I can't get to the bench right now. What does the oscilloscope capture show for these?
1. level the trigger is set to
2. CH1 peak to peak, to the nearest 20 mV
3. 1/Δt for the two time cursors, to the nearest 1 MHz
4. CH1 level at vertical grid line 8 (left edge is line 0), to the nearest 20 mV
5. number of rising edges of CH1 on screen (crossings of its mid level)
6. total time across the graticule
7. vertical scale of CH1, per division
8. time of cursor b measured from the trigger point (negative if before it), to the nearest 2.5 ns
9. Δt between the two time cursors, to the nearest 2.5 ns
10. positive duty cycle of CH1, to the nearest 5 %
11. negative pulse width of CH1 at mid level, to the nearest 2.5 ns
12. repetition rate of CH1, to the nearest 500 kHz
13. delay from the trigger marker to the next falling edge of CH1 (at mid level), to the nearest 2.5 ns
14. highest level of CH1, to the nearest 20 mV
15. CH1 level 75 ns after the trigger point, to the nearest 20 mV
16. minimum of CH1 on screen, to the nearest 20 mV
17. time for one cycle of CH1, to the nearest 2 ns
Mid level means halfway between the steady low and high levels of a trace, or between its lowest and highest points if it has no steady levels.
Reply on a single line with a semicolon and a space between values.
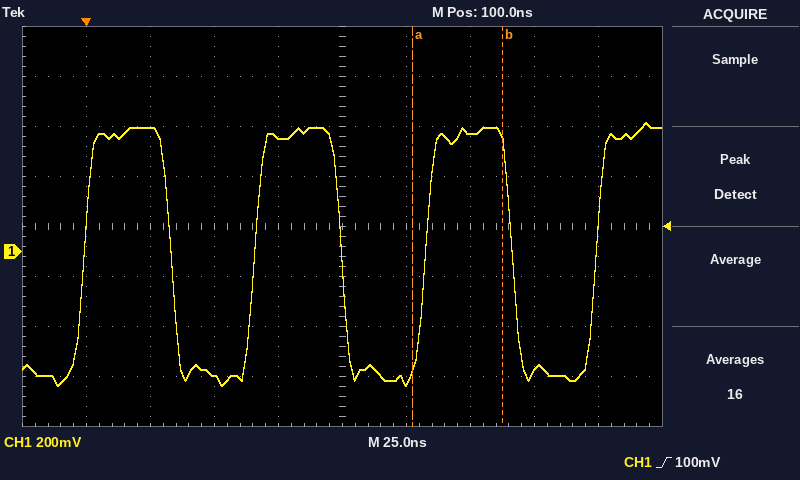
100 mV; 1.06 V; 29 MHz; -480 mV; 4; 250 ns; 200 mV; +162.5 ns; 35.0 ns; 50 %; 32.5 ns; 15.0 MHz; 32.5 ns; 520 mV; 460 mV; -540 mV; 66 ns
